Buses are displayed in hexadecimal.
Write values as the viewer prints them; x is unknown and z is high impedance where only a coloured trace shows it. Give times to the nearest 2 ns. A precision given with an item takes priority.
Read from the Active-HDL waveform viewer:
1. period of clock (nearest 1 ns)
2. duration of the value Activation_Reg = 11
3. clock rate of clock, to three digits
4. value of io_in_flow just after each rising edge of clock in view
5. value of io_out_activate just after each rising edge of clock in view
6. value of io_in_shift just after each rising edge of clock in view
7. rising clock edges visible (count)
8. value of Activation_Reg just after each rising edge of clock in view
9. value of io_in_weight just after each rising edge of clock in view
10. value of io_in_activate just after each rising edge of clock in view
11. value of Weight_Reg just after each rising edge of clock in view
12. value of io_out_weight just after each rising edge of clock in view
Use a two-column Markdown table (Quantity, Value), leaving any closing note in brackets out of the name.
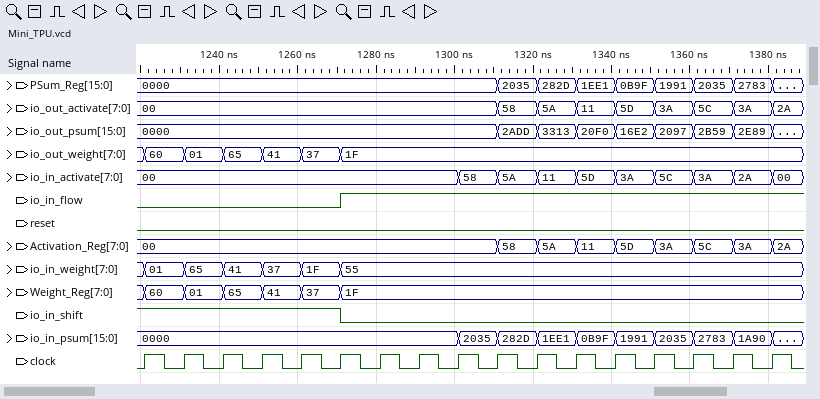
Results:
| Quantity | Value |
|---|---|
| period of clock | 10 ns |
| duration of the value Activation_Reg = 11 | 10 ns |
| clock rate of clock, to three digits | 100 MHz |
| value of io_in_flow just after each rising edge of clock in view | 0 0 0 0 0 1 1 1 1 1 1 1 1 1 1 1 1 |
| value of io_out_activate just after each rising edge of clock in view | 00, 00, 00, 00, 00, 00, 00, 00, 00, 58, 5A, 11, 5D, 3A, 5C, 3A, 2A |
| value of io_in_shift just after each rising edge of clock in view | 1 1 1 1 1 0 0 0 0 0 0 0 0 0 0 0 0 |
| rising clock edges visible | 17 |
| value of Activation_Reg just after each rising edge of clock in view | 00, 00, 00, 00, 00, 00, 00, 00, 00, 58, 5A, 11, 5D, 3A, 5C, 3A, 2A |
| value of io_in_weight just after each rising edge of clock in view | 01, 65, 41, 37, 1F, 55, 55, 55, 55, 55, 55, 55, 55, 55, 55, 55, 55 |
| value of io_in_activate just after each rising edge of clock in view | 00, 00, 00, 00, 00, 00, 00, 00, 58, 5A, 11, 5D, 3A, 5C, 3A, 2A, 00 |
| value of Weight_Reg just after each rising edge of clock in view | 60, 01, 65, 41, 37, 1F, 1F, 1F, 1F, 1F, 1F, 1F, 1F, 1F, 1F, 1F, 1F |
| value of io_out_weight just after each rising edge of clock in view | 60, 01, 65, 41, 37, 1F, 1F, 1F, 1F, 1F, 1F, 1F, 1F, 1F, 1F, 1F, 1F |
